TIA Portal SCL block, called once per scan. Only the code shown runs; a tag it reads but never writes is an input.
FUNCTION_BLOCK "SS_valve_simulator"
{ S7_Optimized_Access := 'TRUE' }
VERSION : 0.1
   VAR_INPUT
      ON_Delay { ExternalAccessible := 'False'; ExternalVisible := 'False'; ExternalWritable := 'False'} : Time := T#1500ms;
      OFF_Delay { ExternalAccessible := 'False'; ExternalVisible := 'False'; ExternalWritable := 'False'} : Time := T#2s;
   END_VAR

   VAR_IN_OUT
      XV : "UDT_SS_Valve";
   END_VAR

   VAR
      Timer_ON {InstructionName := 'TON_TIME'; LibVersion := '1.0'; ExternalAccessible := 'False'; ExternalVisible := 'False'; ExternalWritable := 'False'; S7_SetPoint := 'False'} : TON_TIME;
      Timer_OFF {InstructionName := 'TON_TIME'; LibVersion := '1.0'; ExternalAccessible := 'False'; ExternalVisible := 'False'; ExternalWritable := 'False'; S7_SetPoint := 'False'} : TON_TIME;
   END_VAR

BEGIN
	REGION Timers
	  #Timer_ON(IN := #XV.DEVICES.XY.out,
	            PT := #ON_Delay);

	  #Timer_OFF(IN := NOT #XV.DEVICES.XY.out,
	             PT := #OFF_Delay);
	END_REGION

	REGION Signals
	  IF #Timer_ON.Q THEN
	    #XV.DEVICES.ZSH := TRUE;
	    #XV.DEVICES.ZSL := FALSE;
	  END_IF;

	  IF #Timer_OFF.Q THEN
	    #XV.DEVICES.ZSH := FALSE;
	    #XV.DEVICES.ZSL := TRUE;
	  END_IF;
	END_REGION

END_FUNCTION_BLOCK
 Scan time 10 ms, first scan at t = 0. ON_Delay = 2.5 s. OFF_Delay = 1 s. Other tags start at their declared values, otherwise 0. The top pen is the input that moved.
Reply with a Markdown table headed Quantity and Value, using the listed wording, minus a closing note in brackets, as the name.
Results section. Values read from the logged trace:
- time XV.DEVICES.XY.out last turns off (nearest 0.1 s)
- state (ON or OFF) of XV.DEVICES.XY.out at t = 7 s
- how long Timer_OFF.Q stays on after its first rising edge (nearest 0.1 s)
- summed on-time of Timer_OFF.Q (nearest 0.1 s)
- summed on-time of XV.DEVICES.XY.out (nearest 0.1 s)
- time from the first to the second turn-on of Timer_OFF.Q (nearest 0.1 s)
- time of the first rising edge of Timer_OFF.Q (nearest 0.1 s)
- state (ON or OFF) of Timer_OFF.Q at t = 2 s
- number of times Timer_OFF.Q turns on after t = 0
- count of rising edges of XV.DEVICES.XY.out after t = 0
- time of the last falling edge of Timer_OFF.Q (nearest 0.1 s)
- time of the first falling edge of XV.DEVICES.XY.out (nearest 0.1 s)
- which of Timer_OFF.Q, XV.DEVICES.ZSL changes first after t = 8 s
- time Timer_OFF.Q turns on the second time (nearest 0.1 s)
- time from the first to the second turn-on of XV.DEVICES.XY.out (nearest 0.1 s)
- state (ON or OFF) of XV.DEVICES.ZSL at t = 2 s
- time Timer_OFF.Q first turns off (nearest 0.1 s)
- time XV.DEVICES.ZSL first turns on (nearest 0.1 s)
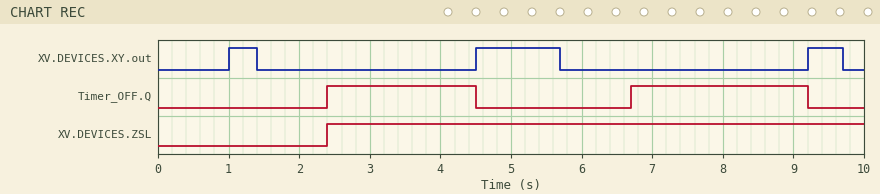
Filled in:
| Quantity | Value |
|---|---|
| time XV.DEVICES.XY.out last turns off | 9.7 s |
| state (ON or OFF) of XV.DEVICES.XY.out at t = 7 s | OFF |
| how long Timer_OFF.Q stays on after its first rising edge | 2.1 s |
| summed on-time of Timer_OFF.Q | 4.6 s |
| summed on-time of XV.DEVICES.XY.out | 2.1 s |
| time from the first to the second turn-on of Timer_OFF.Q | 4.3 s |
| time of the first rising edge of Timer_OFF.Q | 2.4 s |
| state (ON or OFF) of Timer_OFF.Q at t = 2 s | OFF |
| number of times Timer_OFF.Q turns on after t = 0 | 2 |
| count of rising edges of XV.DEVICES.XY.out after t = 0 | 3 |
| time of the last falling edge of Timer_OFF.Q | 9.2 s |
| time of the first falling edge of XV.DEVICES.XY.out | 1.4 s |
| which of Timer_OFF.Q, XV.DEVICES.ZSL changes first after t = 8 s | Timer_OFF.Q |
| time Timer_OFF.Q turns on the second time | 6.7 s |
| time from the first to the second turn-on of XV.DEVICES.XY.out | 3.5 s |
| state (ON or OFF) of XV.DEVICES.ZSL at t = 2 s | OFF |
| time Timer_OFF.Q first turns off | 4.5 s |
| time XV.DEVICES.ZSL first turns on | 2.4 s |
